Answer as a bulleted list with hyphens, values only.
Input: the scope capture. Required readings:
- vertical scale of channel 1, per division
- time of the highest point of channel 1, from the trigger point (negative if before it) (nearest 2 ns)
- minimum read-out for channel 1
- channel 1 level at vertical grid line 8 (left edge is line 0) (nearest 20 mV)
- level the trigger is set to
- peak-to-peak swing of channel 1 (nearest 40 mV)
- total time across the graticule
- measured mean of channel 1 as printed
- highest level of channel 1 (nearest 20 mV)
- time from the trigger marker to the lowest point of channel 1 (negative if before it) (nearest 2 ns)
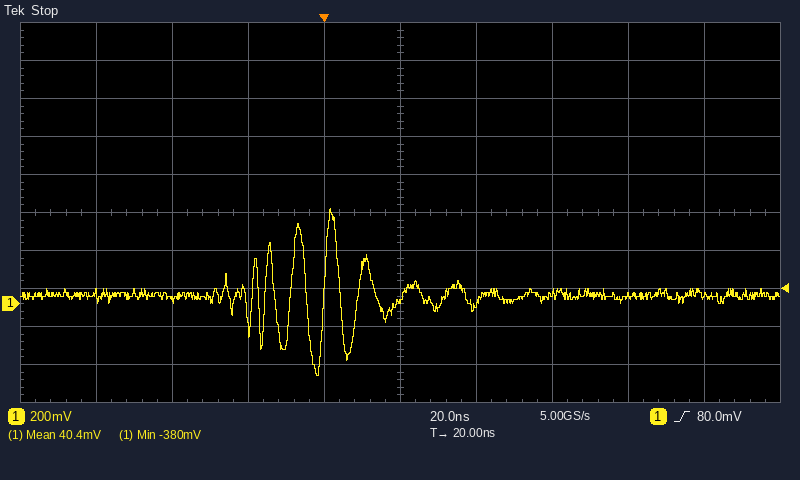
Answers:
- 200 mV
- +2 ns
- -380 mV
- 40 mV
- 80.0 mV
- 880 mV
- 200 ns
- 40.4 mV
- 500 mV
- -2 ns
